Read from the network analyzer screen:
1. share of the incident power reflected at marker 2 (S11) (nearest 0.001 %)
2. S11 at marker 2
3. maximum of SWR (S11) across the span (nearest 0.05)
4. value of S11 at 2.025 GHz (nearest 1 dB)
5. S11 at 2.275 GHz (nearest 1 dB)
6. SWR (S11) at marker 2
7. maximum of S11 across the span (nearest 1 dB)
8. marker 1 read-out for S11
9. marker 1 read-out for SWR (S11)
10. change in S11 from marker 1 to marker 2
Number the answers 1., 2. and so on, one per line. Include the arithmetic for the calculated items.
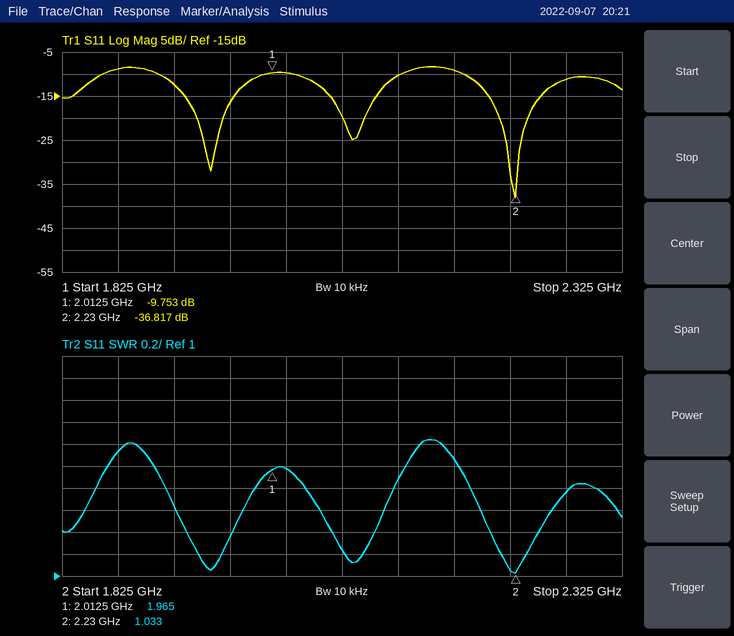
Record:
1. 10^(-36.817/10) ≈ 0.021 %
2. -36.817 dB
3. 2.25
4. -10 dB
5. -11 dB
6. 1.033
7. -8 dB
8. -9.753 dB
9. 1.965
10. -36.817 − (-9.753) = -27.064 dB
